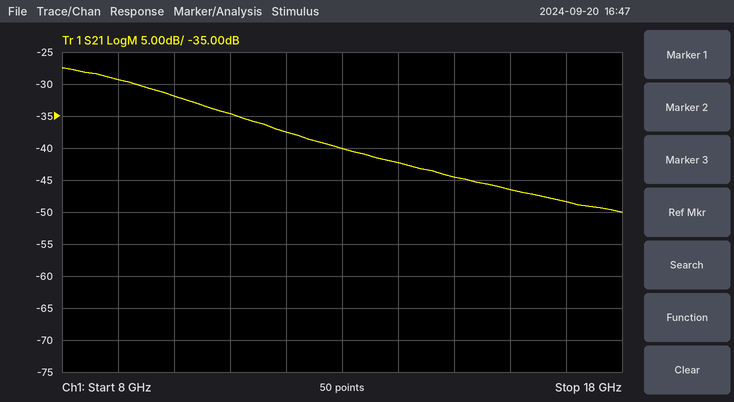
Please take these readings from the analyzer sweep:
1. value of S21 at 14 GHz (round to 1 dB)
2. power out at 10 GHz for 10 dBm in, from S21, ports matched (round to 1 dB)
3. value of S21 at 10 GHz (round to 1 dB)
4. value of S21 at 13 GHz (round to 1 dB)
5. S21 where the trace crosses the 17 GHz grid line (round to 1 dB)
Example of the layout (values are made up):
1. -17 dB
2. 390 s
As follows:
1. -42 dB
2. -22 dBm
3. -32 dB
4. -40 dB
5. -48 dB
